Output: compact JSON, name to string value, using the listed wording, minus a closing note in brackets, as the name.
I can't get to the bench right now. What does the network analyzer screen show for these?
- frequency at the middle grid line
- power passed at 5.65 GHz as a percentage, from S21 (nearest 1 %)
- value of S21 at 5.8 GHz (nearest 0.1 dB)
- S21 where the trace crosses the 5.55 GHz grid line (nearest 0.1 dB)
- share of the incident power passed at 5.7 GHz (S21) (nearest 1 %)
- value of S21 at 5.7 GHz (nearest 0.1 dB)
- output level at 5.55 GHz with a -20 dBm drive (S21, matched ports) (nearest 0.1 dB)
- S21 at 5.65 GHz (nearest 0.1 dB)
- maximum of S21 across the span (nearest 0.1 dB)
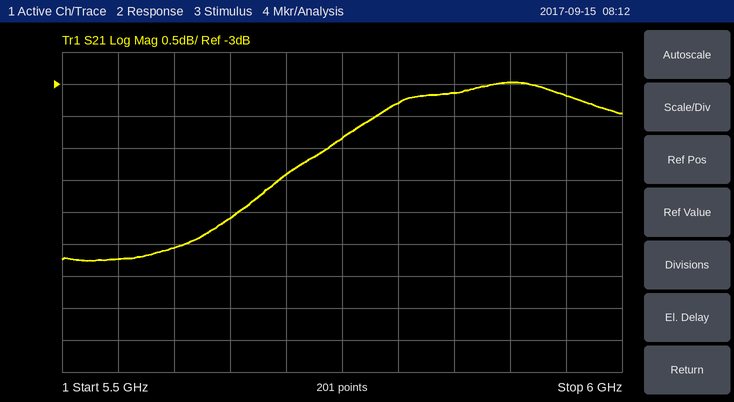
{"frequency at the middle grid line": "5.75 GHz", "power passed at 5.65 GHz as a percentage, from S21": "31 %", "value of S21 at 5.8 GHz": "-3.3 dB", "S21 where the trace crosses the 5.55 GHz grid line": "-5.7 dB", "share of the incident power passed at 5.7 GHz (S21)": "36 %", "value of S21 at 5.7 GHz": "-4.4 dB", "output level at 5.55 GHz with a -20 dBm drive (S21, matched ports)": "-25.7 dBm", "S21 at 5.65 GHz": "-5.1 dB", "maximum of S21 across the span": "-3.0 dB"}
